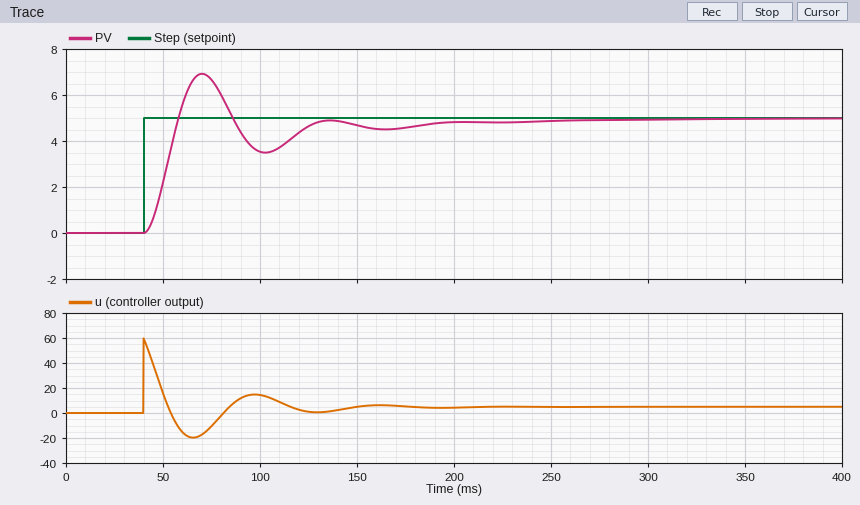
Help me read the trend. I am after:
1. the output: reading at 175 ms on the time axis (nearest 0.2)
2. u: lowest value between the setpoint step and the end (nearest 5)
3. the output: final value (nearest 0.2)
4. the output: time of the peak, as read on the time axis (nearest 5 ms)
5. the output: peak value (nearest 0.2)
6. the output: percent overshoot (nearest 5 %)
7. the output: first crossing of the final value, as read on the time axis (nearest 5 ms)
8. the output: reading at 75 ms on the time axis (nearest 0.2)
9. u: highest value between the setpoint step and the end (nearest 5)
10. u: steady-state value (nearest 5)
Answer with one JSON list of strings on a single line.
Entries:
["4.6", "-20", "5.0", "70 ms", "7.0", "40 %", "60 ms", "6.6", "60", "5"]
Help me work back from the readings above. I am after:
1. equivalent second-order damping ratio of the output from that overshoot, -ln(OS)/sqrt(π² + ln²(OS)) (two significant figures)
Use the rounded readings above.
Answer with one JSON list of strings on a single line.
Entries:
["0.28"]
